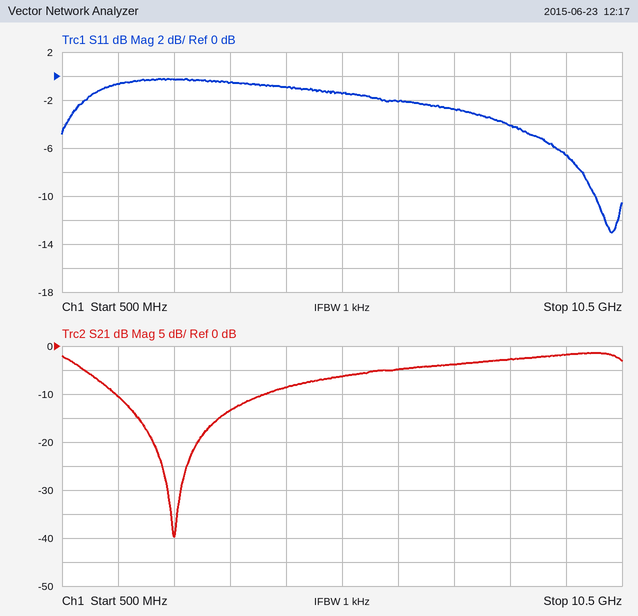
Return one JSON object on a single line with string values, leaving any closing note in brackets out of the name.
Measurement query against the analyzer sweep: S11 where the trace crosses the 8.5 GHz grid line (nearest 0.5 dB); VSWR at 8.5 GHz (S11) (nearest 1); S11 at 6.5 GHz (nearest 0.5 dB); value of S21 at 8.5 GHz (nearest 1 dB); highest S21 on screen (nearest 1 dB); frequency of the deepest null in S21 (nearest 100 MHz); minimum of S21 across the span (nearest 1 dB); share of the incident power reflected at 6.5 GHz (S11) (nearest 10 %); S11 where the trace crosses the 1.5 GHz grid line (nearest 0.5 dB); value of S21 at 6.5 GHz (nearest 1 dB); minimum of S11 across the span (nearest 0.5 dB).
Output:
{"S11 where the trace crosses the 8.5 GHz grid line": "-4.0 dB", "VSWR at 8.5 GHz (S11)": "4", "S11 at 6.5 GHz": "-2.0 dB", "value of S21 at 8.5 GHz": "-3 dB", "highest S21 on screen": "-1 dB", "frequency of the deepest null in S21": "2.5 GHz", "minimum of S21 across the span": "-40 dB", "share of the incident power reflected at 6.5 GHz (S11)": "60 %", "S11 where the trace crosses the 1.5 GHz grid line": "-0.5 dB", "value of S21 at 6.5 GHz": "-5 dB", "minimum of S11 across the span": "-13.0 dB"}
